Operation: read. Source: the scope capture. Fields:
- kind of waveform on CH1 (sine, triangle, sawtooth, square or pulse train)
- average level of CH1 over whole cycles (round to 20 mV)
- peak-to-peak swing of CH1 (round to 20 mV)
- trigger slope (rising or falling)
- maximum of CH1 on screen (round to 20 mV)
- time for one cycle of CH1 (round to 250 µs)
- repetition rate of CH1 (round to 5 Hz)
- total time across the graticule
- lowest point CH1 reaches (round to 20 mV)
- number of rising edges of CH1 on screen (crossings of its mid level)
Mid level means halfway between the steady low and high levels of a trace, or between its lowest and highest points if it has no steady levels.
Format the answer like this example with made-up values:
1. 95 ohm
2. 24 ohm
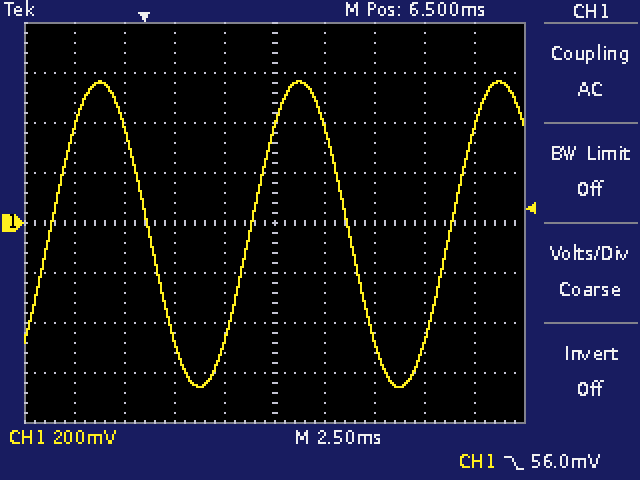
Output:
1. sine
2. -40 mV
3. 1.22 V
4. falling
5. 560 mV
6. 10.00 ms
7. 100 Hz
8. 25 ms
9. -660 mV
10. 3
